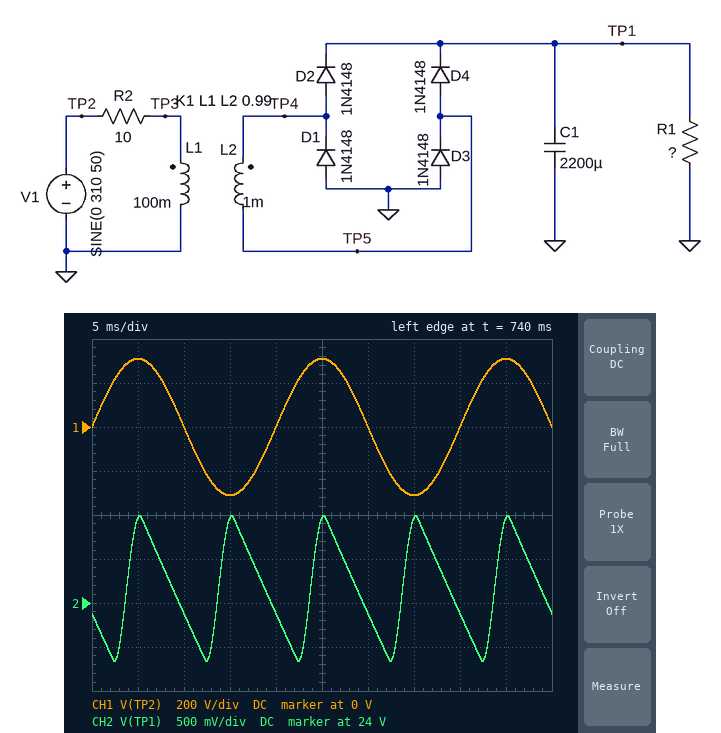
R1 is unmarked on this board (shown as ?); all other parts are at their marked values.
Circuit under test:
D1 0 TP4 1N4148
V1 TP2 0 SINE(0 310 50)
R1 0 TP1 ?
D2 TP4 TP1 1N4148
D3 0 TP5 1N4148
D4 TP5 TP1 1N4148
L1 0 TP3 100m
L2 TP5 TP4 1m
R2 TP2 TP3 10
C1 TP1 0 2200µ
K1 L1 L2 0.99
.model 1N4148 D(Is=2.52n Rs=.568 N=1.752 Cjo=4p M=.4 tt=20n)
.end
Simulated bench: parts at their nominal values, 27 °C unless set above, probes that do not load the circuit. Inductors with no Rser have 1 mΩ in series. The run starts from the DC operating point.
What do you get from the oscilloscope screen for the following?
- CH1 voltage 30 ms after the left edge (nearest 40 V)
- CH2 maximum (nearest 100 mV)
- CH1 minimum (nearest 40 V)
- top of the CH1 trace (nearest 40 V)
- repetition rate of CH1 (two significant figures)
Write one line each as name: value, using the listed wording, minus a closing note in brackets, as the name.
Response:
CH1 voltage 30 ms after the left edge: 0 V
CH2 maximum: 25.0 V
CH1 minimum: -320 V
top of the CH1 trace: 320 V
repetition rate of CH1: 50 Hz
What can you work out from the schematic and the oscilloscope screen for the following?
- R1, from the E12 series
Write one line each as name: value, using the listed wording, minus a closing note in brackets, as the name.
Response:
R1, from the E12 series: 47 Ω
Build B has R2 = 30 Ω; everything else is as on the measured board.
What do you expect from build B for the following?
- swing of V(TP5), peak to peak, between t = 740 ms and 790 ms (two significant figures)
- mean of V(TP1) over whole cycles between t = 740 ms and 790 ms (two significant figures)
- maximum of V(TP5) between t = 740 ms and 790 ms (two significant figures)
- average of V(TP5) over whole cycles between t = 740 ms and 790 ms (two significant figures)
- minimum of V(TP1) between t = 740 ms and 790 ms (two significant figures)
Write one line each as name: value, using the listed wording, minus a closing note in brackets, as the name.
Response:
swing of V(TP5), peak to peak, between t = 740 ms and 790 ms: 22 V
mean of V(TP1) over whole cycles between t = 740 ms and 790 ms: 18 V
maximum of V(TP5) between t = 740 ms and 790 ms: 20 V
average of V(TP5) over whole cycles between t = 740 ms and 790 ms: 8.9 V
minimum of V(TP1) between t = 740 ms and 790 ms: 17 V
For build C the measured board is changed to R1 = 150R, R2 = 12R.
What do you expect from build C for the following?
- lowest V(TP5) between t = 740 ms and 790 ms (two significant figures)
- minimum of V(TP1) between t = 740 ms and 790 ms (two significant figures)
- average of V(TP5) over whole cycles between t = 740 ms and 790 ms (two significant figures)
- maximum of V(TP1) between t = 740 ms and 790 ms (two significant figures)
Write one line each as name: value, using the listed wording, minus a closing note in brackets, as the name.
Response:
lowest V(TP5) between t = 740 ms and 790 ms: -1.6 V
minimum of V(TP1) between t = 740 ms and 790 ms: 25 V
average of V(TP5) over whole cycles between t = 740 ms and 790 ms: 13 V
maximum of V(TP1) between t = 740 ms and 790 ms: 26 V
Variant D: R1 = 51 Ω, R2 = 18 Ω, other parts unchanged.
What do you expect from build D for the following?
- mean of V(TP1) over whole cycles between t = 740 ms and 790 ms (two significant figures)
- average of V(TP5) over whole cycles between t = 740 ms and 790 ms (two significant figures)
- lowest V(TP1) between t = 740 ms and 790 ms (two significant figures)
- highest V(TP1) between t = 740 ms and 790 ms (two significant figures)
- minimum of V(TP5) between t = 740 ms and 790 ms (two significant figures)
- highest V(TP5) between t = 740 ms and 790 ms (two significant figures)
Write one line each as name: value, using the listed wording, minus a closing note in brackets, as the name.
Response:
mean of V(TP1) over whole cycles between t = 740 ms and 790 ms: 22 V
average of V(TP5) over whole cycles between t = 740 ms and 790 ms: 11 V
lowest V(TP1) between t = 740 ms and 790 ms: 21 V
highest V(TP1) between t = 740 ms and 790 ms: 23 V
minimum of V(TP5) between t = 740 ms and 790 ms: -2.1 V
highest V(TP5) between t = 740 ms and 790 ms: 24 V
